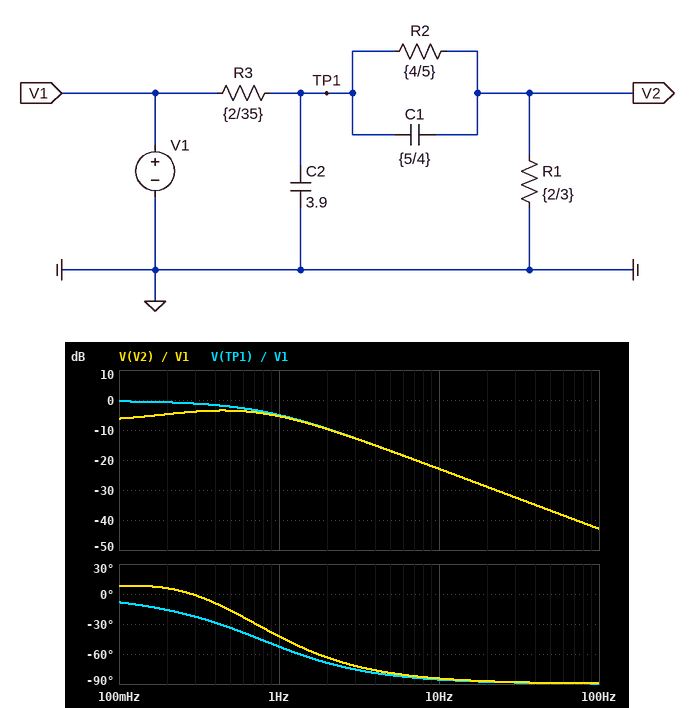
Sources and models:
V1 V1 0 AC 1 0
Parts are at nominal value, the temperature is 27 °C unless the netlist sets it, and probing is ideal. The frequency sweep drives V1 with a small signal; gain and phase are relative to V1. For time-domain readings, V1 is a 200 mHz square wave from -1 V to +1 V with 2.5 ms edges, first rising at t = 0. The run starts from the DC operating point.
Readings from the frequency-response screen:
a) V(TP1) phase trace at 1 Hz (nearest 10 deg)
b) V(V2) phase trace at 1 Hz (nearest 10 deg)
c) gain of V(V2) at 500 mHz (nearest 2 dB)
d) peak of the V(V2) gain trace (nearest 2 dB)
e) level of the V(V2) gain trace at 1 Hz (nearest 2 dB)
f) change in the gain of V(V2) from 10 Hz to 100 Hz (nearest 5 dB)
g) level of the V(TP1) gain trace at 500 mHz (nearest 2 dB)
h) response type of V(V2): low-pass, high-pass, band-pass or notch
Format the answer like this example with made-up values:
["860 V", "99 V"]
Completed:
["-50 deg", "-40 deg", "-4 dB", "-4 dB", "-6 dB", "-20 dB", "-2 dB", "low-pass"]
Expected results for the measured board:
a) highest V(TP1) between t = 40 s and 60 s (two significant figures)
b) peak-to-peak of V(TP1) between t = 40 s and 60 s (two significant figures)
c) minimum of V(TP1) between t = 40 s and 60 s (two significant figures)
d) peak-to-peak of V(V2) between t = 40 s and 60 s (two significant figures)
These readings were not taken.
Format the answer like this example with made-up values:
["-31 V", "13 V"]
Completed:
["960 mV", "1.9 V", "-960 mV", "1.6 V"]
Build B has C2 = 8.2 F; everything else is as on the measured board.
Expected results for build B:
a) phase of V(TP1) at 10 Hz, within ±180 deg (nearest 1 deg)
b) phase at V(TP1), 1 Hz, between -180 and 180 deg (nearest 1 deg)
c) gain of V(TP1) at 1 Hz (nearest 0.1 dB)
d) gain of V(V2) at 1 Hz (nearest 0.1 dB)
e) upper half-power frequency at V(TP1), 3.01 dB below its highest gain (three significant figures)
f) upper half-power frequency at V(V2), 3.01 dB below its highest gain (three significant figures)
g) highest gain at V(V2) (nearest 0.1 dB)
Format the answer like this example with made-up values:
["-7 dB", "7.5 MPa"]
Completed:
["-88 deg", "-70 deg", "-10.0 dB", "-10.4 dB", "337 mHz", "748 mHz", "-5.5 dB"]
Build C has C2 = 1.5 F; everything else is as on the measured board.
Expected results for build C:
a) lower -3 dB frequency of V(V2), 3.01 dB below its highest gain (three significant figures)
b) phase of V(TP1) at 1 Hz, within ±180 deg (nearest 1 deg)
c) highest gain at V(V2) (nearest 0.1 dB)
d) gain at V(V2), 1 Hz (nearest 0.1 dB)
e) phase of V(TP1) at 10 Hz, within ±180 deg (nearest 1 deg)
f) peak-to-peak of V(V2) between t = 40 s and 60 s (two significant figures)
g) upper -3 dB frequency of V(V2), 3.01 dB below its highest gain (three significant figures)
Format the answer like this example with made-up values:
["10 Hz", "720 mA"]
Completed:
["168 mHz", "-27 deg", "-1.9 dB", "-2.1 dB", "-79 deg", "2.1 V", "2.55 Hz"]
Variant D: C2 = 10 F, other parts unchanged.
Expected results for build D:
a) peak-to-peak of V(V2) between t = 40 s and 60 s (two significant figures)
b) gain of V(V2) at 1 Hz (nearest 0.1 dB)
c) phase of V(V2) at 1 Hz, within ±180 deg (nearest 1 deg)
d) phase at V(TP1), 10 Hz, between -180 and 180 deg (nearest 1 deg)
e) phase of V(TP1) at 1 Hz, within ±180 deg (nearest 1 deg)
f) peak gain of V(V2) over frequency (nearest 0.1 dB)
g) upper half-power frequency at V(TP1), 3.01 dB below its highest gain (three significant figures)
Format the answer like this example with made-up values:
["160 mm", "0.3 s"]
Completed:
["1.1 V", "-11.9 dB", "-63 deg", "-88 deg", "-73 deg", "-6.1 dB", "278 mHz"]
